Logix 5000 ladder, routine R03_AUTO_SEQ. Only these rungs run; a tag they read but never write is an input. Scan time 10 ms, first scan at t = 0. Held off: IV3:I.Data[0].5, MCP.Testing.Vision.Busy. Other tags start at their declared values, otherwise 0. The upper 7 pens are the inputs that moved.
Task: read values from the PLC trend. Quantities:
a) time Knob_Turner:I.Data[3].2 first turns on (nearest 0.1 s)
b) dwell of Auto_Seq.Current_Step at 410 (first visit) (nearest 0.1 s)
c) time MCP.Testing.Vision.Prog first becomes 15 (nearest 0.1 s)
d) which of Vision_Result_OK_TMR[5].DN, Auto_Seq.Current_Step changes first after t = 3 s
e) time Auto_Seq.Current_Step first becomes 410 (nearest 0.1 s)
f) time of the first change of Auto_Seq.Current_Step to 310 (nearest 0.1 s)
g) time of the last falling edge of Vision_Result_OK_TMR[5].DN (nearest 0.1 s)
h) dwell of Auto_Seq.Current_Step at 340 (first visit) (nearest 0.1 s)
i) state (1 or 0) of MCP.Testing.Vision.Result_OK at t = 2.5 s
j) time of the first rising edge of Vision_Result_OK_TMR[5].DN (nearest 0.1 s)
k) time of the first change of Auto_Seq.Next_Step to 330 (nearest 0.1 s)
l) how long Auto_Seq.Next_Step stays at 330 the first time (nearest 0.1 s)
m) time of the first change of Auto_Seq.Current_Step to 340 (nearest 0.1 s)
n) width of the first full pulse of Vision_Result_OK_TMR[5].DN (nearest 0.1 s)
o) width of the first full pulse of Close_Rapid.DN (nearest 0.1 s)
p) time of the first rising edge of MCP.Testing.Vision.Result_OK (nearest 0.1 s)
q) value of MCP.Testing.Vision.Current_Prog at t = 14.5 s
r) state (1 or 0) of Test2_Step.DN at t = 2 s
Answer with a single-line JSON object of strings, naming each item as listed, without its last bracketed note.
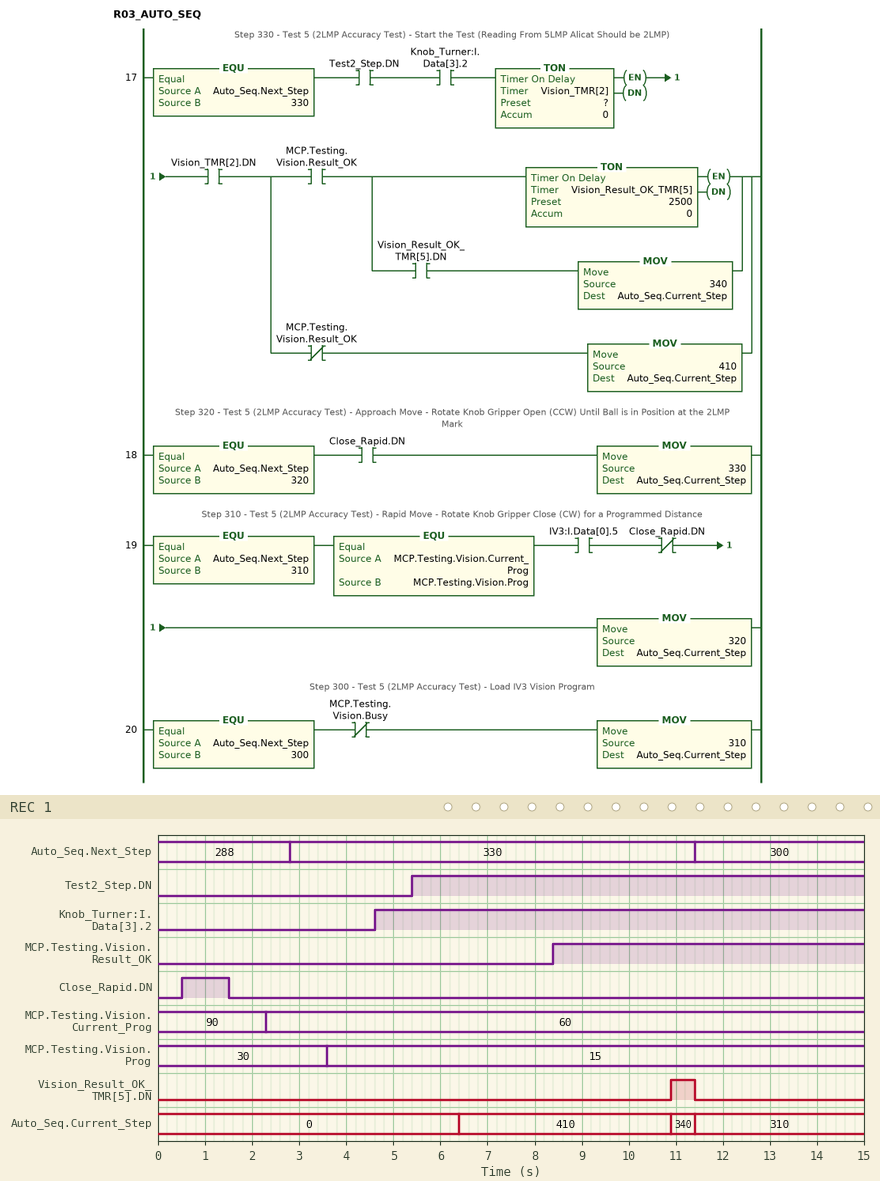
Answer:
{"time Knob_Turner:I.Data[3].2 first turns on": "4.6 s", "dwell of Auto_Seq.Current_Step at 410 (first visit)": "4.5 s", "time MCP.Testing.Vision.Prog first becomes 15": "3.6 s", "which of Vision_Result_OK_TMR[5].DN, Auto_Seq.Current_Step changes first after t = 3 s": "Auto_Seq.Current_Step", "time Auto_Seq.Current_Step first becomes 410": "6.4 s", "time of the first change of Auto_Seq.Current_Step to 310": "11.4 s", "time of the last falling edge of Vision_Result_OK_TMR[5].DN": "11.4 s", "dwell of Auto_Seq.Current_Step at 340 (first visit)": "0.5 s", "state (1 or 0) of MCP.Testing.Vision.Result_OK at t = 2.5 s": "0", "time of the first rising edge of Vision_Result_OK_TMR[5].DN": "10.9 s", "time of the first change of Auto_Seq.Next_Step to 330": "2.8 s", "how long Auto_Seq.Next_Step stays at 330 the first time": "8.6 s", "time of the first change of Auto_Seq.Current_Step to 340": "10.9 s", "width of the first full pulse of Vision_Result_OK_TMR[5].DN": "0.5 s", "width of the first full pulse of Close_Rapid.DN": "1.0 s", "time of the first rising edge of MCP.Testing.Vision.Result_OK": "8.4 s", "value of MCP.Testing.Vision.Current_Prog at t = 14.5 s": "60", "state (1 or 0) of Test2_Step.DN at t = 2 s": "0"}
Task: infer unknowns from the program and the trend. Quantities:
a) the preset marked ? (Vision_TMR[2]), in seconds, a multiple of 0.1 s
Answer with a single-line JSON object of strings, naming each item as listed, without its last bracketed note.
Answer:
{"the preset marked ? (Vision_TMR[2]), in seconds, a multiple of 0.1 s": "1.0 s"}
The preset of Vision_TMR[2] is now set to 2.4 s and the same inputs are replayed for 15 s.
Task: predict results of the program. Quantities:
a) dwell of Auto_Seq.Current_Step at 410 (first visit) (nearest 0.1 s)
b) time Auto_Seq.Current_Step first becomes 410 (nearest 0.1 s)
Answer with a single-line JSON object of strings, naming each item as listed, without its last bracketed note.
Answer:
{"dwell of Auto_Seq.Current_Step at 410 (first visit)": "3.1 s", "time Auto_Seq.Current_Step first becomes 410": "7.8 s"}
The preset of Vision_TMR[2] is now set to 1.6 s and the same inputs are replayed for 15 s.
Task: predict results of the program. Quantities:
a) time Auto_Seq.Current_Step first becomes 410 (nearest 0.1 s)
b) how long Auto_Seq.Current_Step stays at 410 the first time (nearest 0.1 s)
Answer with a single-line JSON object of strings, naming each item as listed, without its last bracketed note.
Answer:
{"time Auto_Seq.Current_Step first becomes 410": "7.0 s", "how long Auto_Seq.Current_Step stays at 410 the first time": "3.9 s"}
